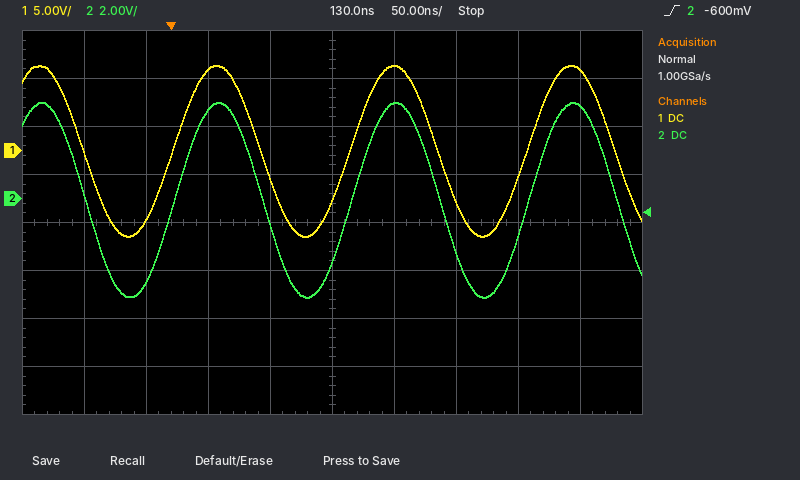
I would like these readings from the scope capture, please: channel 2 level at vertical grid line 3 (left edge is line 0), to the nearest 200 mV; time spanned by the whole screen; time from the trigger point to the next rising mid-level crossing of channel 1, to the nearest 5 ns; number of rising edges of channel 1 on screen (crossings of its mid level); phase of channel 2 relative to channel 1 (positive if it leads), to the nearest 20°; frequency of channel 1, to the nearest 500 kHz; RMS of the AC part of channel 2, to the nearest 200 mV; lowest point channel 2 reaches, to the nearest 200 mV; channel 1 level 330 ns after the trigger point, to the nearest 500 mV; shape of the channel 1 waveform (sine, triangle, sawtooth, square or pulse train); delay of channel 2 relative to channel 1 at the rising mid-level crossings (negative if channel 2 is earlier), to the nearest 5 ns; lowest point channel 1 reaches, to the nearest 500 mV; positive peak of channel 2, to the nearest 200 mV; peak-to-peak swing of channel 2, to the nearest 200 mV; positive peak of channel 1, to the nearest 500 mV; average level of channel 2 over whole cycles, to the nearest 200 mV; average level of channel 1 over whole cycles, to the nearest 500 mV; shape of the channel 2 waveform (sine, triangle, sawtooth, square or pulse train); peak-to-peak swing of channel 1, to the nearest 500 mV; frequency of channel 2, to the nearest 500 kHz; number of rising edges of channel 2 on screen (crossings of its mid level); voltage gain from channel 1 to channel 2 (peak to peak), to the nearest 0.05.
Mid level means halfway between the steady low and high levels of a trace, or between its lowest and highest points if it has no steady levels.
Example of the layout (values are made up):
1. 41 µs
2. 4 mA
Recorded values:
1. 3.6 V
2. 500 ns
3. 145 ns
4. 3
5. 0°
6. 7.0 MHz
7. 2.8 V
8. -4.2 V
9. 8.5 V
10. sine
11. 0 ns
12. -9.0 V
13. 4.0 V
14. 8.2 V
15. 9.0 V
16. 0.0 V
17. 0.0 V
18. sine
19. 18.0 V
20. 7.0 MHz
21. 3
22. 0.45
